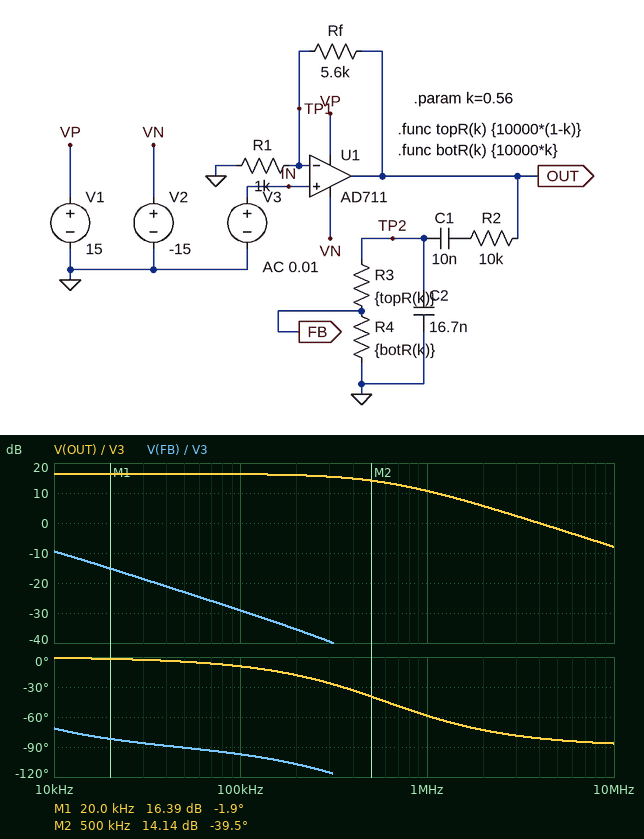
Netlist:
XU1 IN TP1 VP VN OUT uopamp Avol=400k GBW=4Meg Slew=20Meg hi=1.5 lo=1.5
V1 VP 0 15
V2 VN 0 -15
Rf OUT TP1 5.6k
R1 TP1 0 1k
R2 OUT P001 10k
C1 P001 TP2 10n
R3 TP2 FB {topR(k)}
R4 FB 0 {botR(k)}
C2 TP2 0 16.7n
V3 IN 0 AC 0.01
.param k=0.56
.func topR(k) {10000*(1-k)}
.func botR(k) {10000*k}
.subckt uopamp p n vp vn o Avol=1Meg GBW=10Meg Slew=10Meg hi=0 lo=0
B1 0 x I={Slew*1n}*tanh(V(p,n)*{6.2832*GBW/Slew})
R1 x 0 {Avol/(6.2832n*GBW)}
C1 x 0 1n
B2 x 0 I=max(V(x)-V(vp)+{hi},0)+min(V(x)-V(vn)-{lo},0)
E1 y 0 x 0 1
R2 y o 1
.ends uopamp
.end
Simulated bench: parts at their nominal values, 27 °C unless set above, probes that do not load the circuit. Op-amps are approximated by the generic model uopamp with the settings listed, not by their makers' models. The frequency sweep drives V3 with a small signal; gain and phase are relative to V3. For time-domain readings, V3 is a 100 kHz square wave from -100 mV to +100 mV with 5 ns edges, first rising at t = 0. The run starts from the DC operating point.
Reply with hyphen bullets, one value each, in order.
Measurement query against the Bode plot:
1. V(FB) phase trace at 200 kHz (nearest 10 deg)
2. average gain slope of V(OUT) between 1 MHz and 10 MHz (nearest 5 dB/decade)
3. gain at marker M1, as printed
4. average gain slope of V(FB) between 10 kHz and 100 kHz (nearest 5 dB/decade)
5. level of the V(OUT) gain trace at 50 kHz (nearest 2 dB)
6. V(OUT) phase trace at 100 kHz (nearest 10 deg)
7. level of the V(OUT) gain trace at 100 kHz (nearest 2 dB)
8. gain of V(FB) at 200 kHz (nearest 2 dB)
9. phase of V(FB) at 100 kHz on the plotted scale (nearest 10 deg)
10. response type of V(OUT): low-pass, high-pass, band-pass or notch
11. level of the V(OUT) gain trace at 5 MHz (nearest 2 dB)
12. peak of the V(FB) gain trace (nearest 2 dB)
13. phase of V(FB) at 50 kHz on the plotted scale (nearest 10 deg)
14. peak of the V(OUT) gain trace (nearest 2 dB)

- -110 deg
- -20 dB/decade
- 16.39 dB
- -20 dB/decade
- 16 dB
- -10 deg
- 16 dB
- -36 dB
- -100 deg
- low-pass
- -2 dB
- -10 dB
- -90 deg
- 16 dB
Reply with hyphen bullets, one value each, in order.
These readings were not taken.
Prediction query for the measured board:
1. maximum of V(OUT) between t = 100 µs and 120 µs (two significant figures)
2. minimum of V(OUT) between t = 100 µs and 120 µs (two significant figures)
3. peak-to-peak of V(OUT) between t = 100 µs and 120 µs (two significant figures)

- 660 mV
- -660 mV
- 1.3 V
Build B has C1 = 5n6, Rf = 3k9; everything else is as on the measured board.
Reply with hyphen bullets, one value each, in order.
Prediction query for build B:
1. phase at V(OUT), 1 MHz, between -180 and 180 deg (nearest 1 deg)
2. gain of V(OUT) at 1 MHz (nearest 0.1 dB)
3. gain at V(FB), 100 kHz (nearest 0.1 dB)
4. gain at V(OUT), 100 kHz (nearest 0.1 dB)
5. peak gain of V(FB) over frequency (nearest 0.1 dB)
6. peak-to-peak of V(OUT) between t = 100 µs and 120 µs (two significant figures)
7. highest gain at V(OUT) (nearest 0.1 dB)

- -51 deg
- 9.8 dB
- -31.7 dB
- 13.7 dB
- -5.2 dB
- 980 mV
- 13.8 dB
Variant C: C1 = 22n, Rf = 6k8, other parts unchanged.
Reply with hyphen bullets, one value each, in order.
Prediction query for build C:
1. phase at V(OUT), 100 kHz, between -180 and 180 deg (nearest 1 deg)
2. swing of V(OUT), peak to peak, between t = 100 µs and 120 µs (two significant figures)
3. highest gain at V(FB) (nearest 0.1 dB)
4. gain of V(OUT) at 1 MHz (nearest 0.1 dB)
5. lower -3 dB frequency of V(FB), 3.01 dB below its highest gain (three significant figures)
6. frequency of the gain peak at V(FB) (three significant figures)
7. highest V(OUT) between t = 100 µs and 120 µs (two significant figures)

- -11 deg
- 1.6 V
- 4.0 dB
- 11.0 dB
- 240 Hz
- 830 Hz
- 780 mV
